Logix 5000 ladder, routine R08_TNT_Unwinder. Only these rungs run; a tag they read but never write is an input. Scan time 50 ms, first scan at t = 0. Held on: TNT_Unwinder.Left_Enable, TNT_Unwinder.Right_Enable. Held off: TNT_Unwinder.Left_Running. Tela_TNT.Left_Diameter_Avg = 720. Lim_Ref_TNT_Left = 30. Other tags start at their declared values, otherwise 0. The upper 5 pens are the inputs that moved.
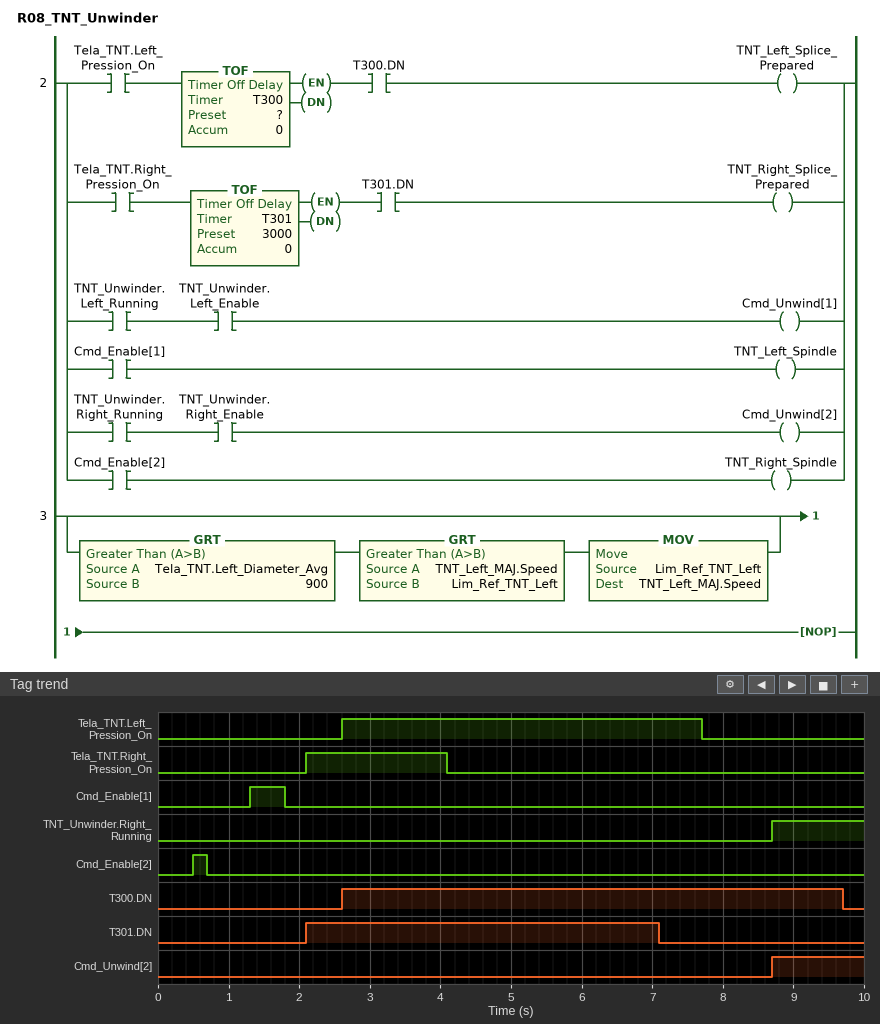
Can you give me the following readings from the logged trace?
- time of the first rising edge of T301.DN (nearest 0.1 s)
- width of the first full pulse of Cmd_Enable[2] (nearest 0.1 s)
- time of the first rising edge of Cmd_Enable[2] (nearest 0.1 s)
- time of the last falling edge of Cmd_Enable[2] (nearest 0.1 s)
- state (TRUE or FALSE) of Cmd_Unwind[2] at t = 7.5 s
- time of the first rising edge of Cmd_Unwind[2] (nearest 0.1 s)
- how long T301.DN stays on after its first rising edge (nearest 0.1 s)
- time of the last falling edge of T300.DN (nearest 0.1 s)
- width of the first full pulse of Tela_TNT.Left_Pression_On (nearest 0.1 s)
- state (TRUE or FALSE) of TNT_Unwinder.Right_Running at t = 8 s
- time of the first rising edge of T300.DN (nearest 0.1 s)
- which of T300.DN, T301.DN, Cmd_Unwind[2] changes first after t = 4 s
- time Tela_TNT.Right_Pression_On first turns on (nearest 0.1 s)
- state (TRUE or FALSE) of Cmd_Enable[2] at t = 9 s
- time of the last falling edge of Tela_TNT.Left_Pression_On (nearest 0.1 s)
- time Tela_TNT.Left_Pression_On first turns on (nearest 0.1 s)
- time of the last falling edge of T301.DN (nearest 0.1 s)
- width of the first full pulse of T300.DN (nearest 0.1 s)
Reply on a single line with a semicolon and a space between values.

2.1 s; 0.2 s; 0.5 s; 0.7 s; FALSE; 8.7 s; 5.0 s; 9.7 s; 5.1 s; FALSE; 2.6 s; T301.DN; 2.1 s; FALSE; 7.7 s; 2.6 s; 7.1 s; 7.1 s
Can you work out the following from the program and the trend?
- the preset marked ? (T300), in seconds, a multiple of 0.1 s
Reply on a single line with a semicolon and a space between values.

2.0 s
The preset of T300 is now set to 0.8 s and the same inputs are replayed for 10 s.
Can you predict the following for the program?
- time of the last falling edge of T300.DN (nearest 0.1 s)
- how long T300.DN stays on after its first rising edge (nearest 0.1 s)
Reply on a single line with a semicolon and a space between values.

8.5 s; 5.9 s
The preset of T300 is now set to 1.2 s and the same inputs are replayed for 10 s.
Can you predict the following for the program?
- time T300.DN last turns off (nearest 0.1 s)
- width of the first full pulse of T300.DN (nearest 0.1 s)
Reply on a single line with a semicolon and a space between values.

8.9 s; 6.3 s
